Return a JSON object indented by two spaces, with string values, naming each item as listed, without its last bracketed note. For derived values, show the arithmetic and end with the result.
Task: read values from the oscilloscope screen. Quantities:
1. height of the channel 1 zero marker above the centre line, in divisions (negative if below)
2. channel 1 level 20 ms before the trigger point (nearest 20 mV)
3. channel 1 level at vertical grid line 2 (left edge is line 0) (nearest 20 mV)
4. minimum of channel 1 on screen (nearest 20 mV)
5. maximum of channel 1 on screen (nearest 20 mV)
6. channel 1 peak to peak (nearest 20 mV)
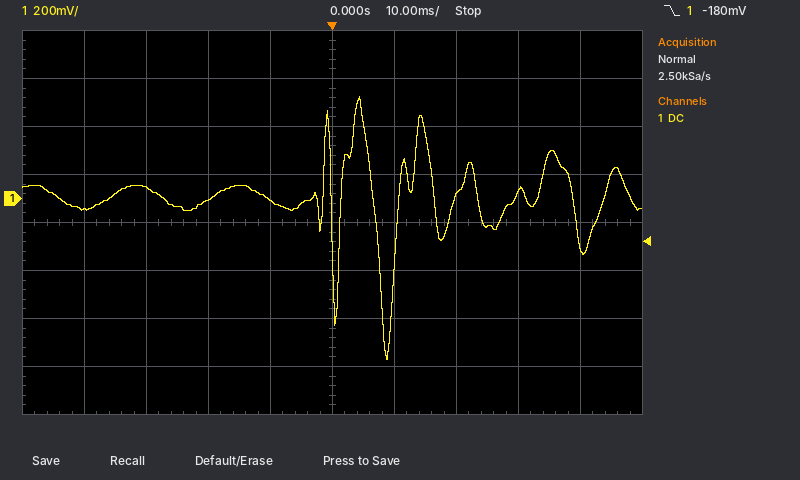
{
  "height of the channel 1 zero marker above the centre line, in divisions": "+0.5 div",
  "channel 1 level 20 ms before the trigger point": "0 mV",
  "channel 1 level at vertical grid line 2 (left edge is line 0)": "40 mV",
  "minimum of channel 1 on screen": "-680 mV",
  "maximum of channel 1 on screen": "420 mV",
  "channel 1 peak to peak": "420 mV − (-680 mV) = 1.10 V"
}
